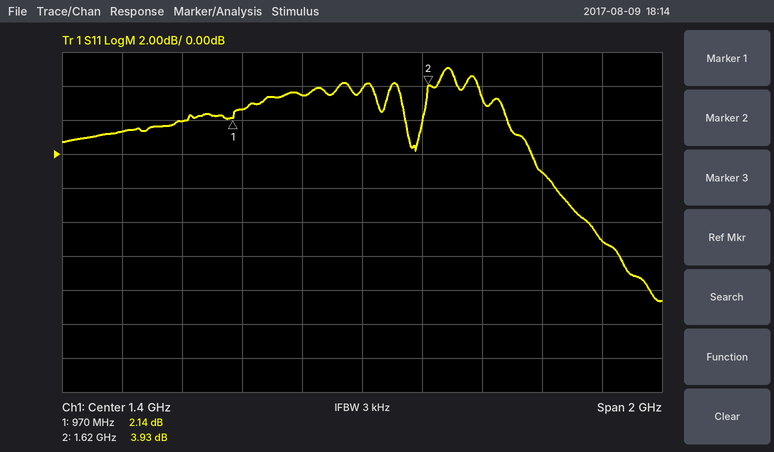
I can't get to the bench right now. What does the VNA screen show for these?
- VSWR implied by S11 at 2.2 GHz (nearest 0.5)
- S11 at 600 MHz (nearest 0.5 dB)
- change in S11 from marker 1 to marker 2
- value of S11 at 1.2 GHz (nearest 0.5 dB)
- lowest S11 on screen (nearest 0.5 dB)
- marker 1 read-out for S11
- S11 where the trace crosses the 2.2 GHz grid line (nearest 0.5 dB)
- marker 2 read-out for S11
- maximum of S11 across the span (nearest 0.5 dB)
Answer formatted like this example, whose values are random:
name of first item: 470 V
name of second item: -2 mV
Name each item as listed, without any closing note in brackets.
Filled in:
VSWR implied by S11 at 2.2 GHz: 3.5
S11 at 600 MHz: 1.5 dB
change in S11 from marker 1 to marker 2: 1.79 dB
value of S11 at 1.2 GHz: 3.5 dB
lowest S11 on screen: -8.5 dB
marker 1 read-out for S11: 2.14 dB
S11 where the trace crosses the 2.2 GHz grid line: -5.0 dB
marker 2 read-out for S11: 3.93 dB
maximum of S11 across the span: 5.0 dB
